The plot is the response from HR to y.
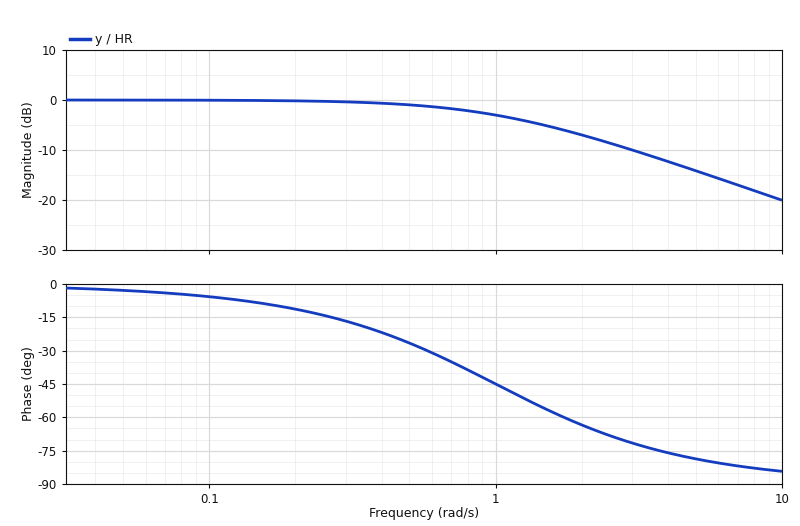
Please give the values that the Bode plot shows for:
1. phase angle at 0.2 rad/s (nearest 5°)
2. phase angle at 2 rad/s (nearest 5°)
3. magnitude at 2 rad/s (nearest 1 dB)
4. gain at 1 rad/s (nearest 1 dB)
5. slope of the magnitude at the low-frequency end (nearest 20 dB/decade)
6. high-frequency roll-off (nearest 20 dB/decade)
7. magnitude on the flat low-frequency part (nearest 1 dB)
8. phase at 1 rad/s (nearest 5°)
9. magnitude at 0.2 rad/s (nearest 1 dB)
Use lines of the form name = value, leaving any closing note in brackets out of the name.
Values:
phase angle at 0.2 rad/s = -10°
phase angle at 2 rad/s = -65°
magnitude at 2 rad/s = -7 dB
gain at 1 rad/s = -3 dB
slope of the magnitude at the low-frequency end = 0 dB/decade
high-frequency roll-off = -20 dB/decade
magnitude on the flat low-frequency part = 0 dB
phase at 1 rad/s = -45°
magnitude at 0.2 rad/s = 0 dB
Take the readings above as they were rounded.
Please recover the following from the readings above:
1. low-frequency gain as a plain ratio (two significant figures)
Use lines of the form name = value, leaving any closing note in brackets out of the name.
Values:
low-frequency gain as a plain ratio = 1.0
